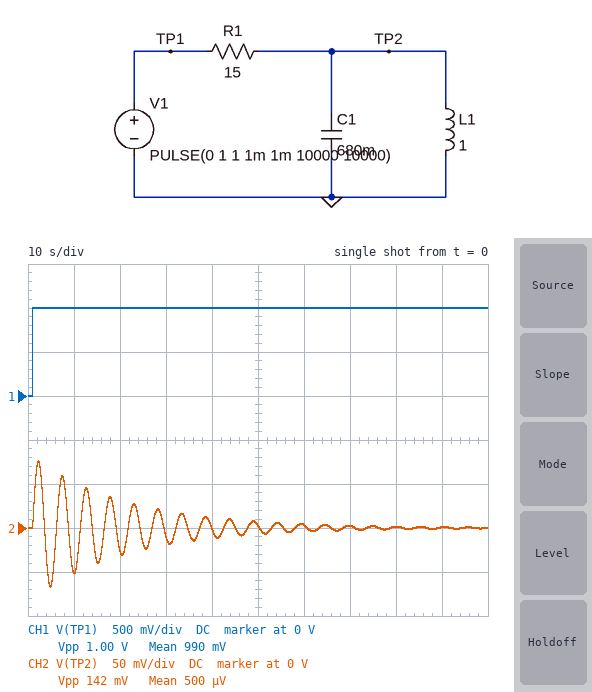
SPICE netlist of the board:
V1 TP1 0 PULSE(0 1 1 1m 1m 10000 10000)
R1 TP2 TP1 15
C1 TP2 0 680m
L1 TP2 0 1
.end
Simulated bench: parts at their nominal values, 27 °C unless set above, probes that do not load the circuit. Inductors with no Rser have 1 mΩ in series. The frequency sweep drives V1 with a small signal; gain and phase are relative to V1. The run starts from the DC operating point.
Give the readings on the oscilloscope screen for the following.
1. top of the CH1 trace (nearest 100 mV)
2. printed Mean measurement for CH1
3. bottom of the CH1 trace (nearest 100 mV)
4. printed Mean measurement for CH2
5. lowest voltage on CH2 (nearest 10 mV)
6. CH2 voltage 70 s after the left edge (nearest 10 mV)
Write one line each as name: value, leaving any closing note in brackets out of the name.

top of the CH1 trace: 1.0 V
printed Mean measurement for CH1: 990 mV
bottom of the CH1 trace: 0 V
printed Mean measurement for CH2: 500 µV
lowest voltage on CH2: -70 mV
CH2 voltage 70 s after the left edge: 0 V
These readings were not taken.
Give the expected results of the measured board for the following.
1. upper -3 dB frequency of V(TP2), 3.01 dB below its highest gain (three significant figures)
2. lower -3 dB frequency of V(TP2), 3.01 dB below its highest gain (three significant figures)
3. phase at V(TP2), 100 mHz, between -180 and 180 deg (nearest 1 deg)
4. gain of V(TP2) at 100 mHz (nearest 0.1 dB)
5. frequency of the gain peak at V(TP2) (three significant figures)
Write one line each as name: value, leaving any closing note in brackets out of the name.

upper -3 dB frequency of V(TP2), 3.01 dB below its highest gain: 201 mHz
lower -3 dB frequency of V(TP2), 3.01 dB below its highest gain: 185 mHz
phase at V(TP2), 100 mHz, between -180 and 180 deg: 87 deg
gain of V(TP2) at 100 mHz: -24.9 dB
frequency of the gain peak at V(TP2): 193 mHz
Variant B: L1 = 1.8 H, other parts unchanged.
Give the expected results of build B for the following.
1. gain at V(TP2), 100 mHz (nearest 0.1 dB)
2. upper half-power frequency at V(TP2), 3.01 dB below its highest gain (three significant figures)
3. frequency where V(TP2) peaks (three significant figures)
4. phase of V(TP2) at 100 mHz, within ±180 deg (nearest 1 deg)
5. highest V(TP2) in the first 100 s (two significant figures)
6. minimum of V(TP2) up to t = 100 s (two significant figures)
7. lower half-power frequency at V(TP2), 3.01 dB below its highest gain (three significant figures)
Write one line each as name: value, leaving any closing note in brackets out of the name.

gain at V(TP2), 100 mHz: -16.8 dB
upper half-power frequency at V(TP2), 3.01 dB below its highest gain: 152 mHz
frequency where V(TP2) peaks: 144 mHz
phase of V(TP2) at 100 mHz, within ±180 deg: 82 deg
highest V(TP2) in the first 100 s: 100 mV
minimum of V(TP2) up to t = 100 s: -84 mV
lower half-power frequency at V(TP2), 3.01 dB below its highest gain: 136 mHz
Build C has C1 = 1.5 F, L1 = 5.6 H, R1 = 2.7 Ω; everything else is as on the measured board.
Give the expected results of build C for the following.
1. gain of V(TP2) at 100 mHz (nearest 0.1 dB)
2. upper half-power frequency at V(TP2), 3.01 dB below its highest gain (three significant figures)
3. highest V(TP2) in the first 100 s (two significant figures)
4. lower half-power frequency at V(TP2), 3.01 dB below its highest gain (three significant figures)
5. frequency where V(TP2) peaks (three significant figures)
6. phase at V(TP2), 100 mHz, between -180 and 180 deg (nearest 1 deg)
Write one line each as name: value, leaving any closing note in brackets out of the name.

gain of V(TP2) at 100 mHz: -6.2 dB
upper half-power frequency at V(TP2), 3.01 dB below its highest gain: 78.0 mHz
highest V(TP2) in the first 100 s: 450 mV
lower half-power frequency at V(TP2), 3.01 dB below its highest gain: 38.7 mHz
frequency where V(TP2) peaks: 54.9 mHz
phase at V(TP2), 100 mHz, between -180 and 180 deg: -61 deg
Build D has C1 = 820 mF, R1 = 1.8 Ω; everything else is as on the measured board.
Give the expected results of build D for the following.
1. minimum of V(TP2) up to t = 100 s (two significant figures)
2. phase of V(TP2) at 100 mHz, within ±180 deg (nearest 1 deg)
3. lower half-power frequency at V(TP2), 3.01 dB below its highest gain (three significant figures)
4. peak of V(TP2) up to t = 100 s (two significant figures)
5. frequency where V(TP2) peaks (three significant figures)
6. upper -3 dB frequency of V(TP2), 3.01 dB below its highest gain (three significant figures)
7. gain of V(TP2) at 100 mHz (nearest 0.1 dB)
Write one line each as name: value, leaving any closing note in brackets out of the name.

minimum of V(TP2) up to t = 100 s: -150 mV
phase of V(TP2) at 100 mHz, within ±180 deg: 63 deg
lower half-power frequency at V(TP2), 3.01 dB below its highest gain: 130 mHz
peak of V(TP2) up to t = 100 s: 410 mV
frequency where V(TP2) peaks: 176 mHz
upper -3 dB frequency of V(TP2), 3.01 dB below its highest gain: 238 mHz
gain of V(TP2) at 100 mHz: -6.8 dB
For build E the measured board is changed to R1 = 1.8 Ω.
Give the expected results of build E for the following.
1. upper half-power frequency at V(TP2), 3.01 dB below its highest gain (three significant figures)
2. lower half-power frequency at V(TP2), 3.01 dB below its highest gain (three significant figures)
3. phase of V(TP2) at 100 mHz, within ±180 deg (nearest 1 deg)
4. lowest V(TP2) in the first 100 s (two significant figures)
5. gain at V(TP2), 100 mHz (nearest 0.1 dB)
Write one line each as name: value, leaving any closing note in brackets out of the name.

upper half-power frequency at V(TP2), 3.01 dB below its highest gain: 269 mHz
lower half-power frequency at V(TP2), 3.01 dB below its highest gain: 139 mHz
phase of V(TP2) at 100 mHz, within ±180 deg: 64 deg
lowest V(TP2) in the first 100 s: -140 mV
gain at V(TP2), 100 mHz: -7.3 dB
